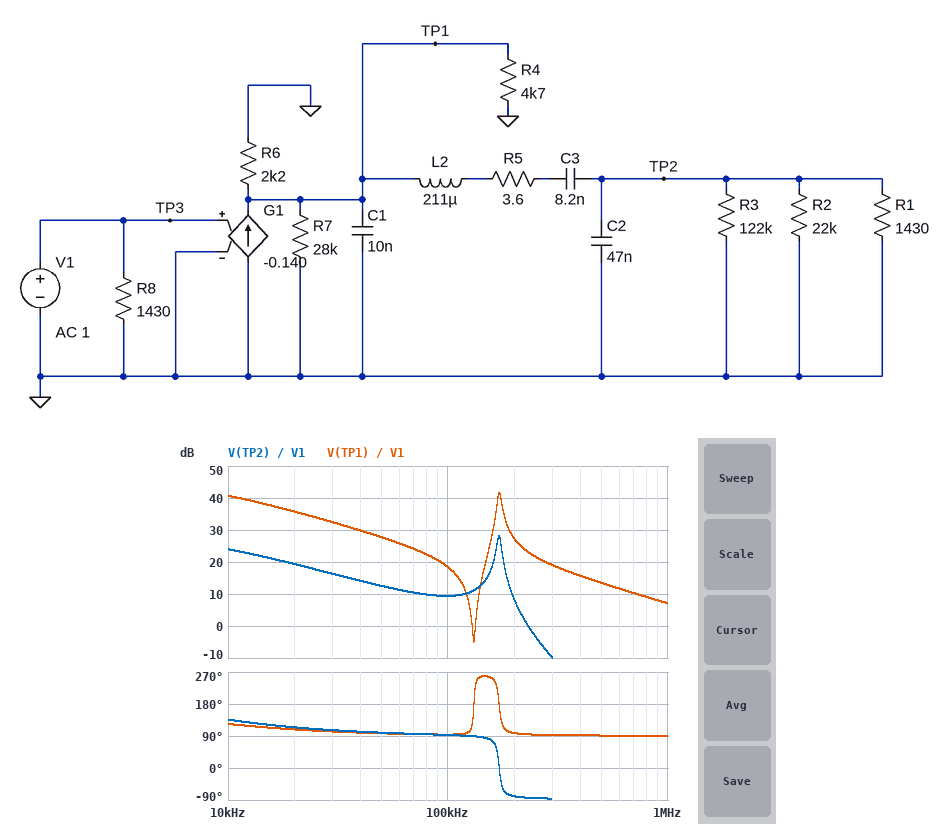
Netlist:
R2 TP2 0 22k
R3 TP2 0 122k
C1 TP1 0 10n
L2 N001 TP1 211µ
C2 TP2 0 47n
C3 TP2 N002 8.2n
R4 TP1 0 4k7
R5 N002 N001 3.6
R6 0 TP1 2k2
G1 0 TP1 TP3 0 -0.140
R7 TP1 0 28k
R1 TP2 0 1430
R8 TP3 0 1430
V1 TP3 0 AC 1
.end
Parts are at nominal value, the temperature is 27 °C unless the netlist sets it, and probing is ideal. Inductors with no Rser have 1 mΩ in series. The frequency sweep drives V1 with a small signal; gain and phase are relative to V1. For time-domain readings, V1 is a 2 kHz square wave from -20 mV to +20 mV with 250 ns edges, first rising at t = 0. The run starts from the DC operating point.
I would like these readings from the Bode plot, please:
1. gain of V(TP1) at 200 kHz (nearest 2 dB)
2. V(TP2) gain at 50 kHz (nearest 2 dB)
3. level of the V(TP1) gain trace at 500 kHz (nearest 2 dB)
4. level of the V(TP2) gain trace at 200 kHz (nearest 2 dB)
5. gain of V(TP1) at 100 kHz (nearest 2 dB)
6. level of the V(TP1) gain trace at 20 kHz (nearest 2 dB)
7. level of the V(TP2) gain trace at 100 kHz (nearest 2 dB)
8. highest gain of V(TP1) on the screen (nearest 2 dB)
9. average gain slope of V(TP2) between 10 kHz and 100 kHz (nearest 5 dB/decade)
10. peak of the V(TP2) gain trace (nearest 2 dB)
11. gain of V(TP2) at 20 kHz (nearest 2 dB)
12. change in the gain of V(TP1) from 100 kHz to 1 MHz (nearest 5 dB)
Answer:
28 dB
12 dB
14 dB
8 dB
18 dB
36 dB
10 dB
42 dB
-15 dB/decade
28 dB
20 dB
-10 dB
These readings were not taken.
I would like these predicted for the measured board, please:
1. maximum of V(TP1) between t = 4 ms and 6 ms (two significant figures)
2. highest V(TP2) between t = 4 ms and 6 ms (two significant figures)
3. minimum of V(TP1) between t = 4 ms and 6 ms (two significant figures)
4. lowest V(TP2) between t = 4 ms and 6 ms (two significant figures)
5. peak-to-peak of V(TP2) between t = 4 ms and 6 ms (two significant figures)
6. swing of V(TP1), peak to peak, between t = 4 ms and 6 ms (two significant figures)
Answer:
4.0 V
660 mV
-4.0 V
-660 mV
1.3 V
7.9 V
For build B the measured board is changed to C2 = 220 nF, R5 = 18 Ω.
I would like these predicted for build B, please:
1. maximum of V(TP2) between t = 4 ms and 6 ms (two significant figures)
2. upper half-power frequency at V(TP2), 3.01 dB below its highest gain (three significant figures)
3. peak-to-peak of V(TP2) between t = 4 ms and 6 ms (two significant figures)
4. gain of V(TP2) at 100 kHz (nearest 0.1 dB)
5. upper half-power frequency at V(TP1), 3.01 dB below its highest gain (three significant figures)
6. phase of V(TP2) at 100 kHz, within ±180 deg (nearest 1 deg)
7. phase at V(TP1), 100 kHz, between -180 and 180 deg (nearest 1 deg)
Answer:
150 mV
7.25 kHz
310 mV
-3.1 dB
6.22 kHz
88 deg
102 deg
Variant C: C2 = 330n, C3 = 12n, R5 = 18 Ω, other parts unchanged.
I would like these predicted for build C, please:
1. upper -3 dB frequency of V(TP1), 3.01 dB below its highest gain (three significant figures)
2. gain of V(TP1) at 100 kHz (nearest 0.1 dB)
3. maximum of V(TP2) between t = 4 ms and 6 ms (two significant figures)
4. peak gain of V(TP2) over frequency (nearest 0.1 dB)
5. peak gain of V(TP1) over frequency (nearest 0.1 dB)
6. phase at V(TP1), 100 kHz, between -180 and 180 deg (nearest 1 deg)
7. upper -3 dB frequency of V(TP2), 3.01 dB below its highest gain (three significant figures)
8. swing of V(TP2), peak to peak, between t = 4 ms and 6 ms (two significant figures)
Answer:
5.15 kHz
7.9 dB
140 mV
16.3 dB
46.0 dB
159 deg
5.86 kHz
280 mV
